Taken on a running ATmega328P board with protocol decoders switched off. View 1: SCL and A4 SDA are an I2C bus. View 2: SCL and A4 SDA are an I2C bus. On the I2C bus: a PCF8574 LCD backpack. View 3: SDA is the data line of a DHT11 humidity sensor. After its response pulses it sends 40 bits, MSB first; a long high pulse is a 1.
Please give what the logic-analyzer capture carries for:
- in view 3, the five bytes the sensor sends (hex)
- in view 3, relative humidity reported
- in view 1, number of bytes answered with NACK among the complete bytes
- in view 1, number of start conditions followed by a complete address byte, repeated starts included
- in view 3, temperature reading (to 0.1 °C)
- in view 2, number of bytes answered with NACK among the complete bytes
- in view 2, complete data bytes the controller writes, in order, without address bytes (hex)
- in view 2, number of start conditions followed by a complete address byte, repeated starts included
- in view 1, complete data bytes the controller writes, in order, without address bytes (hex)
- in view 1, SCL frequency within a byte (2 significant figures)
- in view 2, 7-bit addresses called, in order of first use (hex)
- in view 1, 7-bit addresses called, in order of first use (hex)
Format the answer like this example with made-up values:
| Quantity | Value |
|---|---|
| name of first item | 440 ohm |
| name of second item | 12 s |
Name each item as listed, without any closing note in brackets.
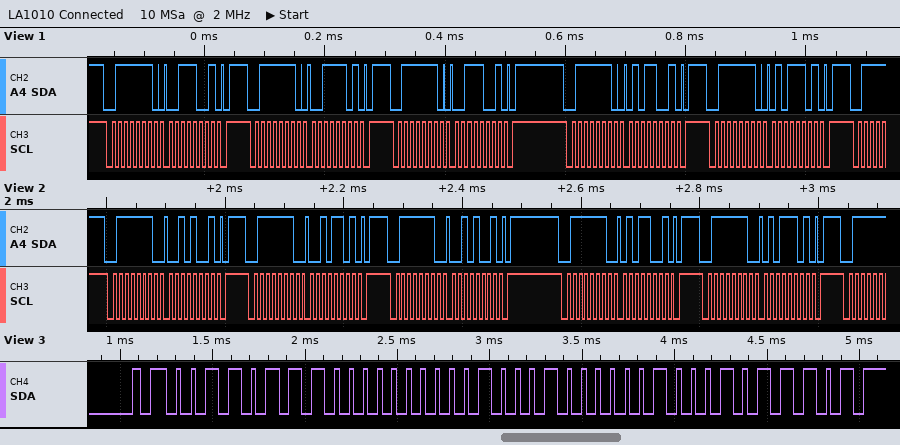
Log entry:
| Quantity | Value |
|---|---|
| in view 3, the five bytes the sensor sends | 37 00 22 04 5D |
| in view 3, relative humidity reported | 55 % |
| in view 1, number of bytes answered with NACK among the complete bytes | 0 |
| in view 1, number of start conditions followed by a complete address byte, repeated starts included | 5 |
| in view 3, temperature reading | 34.4 °C |
| in view 2, number of bytes answered with NACK among the complete bytes | 0 |
| in view 2, complete data bytes the controller writes, in order, without address bytes | 29 2D 29 59 5D |
| in view 2, number of start conditions followed by a complete address byte, repeated starts included | 5 |
| in view 1, complete data bytes the controller writes, in order, without address bytes | 39 3D 39 59 5D |
| in view 1, SCL frequency within a byte | 100 kHz |
| in view 2, 7-bit addresses called, in order of first use | 0x3F |
| in view 1, 7-bit addresses called, in order of first use | 0x3F |
